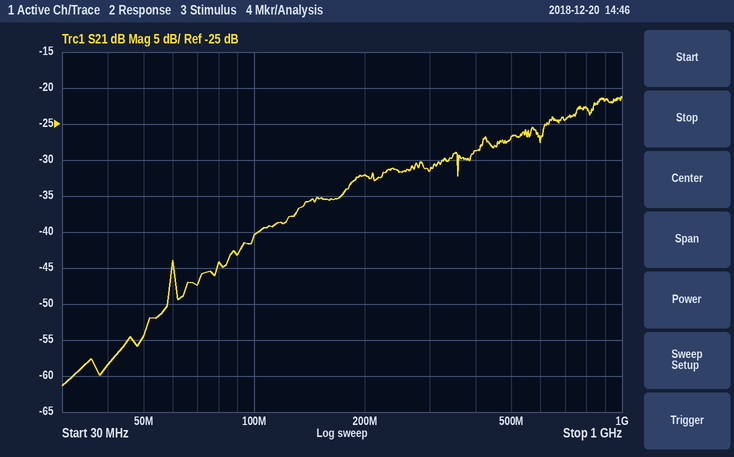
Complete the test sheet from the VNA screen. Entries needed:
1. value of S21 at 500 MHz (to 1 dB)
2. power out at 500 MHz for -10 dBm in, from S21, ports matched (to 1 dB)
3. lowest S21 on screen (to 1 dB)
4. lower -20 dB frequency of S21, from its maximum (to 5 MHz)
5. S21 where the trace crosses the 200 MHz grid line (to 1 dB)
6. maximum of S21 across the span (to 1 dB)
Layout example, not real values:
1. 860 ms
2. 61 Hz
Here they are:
1. -27 dB
2. -37 dBm
3. -61 dB
4. 100 MHz
5. -32 dB
6. -21 dB
